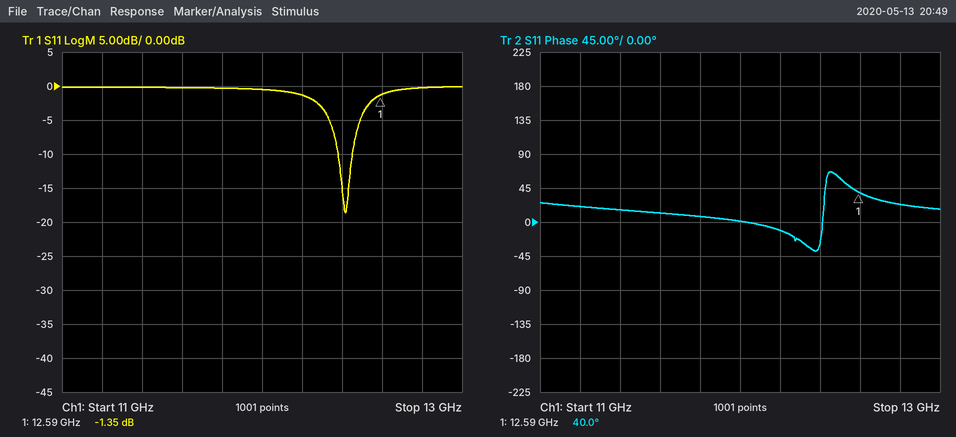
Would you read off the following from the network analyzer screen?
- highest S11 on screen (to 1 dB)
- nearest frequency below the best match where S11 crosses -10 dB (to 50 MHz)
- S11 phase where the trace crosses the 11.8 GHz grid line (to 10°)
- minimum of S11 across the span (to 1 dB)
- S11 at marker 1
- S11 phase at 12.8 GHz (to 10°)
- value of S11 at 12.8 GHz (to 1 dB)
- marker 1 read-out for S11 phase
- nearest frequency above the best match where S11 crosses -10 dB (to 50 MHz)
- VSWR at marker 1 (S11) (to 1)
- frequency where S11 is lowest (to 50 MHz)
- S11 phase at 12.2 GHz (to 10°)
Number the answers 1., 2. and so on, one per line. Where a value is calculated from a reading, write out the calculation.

1. 0 dB
2. 12.40 GHz
3. 10°
4. -19 dB
5. -1.35 dB
6. 20°
7. 0 dB
8. 40.0°
9. 12.45 GHz
10. (1 + 0.8561)/(1 − 0.8561) ≈ 13
11. 12.40 GHz
12. -10°
